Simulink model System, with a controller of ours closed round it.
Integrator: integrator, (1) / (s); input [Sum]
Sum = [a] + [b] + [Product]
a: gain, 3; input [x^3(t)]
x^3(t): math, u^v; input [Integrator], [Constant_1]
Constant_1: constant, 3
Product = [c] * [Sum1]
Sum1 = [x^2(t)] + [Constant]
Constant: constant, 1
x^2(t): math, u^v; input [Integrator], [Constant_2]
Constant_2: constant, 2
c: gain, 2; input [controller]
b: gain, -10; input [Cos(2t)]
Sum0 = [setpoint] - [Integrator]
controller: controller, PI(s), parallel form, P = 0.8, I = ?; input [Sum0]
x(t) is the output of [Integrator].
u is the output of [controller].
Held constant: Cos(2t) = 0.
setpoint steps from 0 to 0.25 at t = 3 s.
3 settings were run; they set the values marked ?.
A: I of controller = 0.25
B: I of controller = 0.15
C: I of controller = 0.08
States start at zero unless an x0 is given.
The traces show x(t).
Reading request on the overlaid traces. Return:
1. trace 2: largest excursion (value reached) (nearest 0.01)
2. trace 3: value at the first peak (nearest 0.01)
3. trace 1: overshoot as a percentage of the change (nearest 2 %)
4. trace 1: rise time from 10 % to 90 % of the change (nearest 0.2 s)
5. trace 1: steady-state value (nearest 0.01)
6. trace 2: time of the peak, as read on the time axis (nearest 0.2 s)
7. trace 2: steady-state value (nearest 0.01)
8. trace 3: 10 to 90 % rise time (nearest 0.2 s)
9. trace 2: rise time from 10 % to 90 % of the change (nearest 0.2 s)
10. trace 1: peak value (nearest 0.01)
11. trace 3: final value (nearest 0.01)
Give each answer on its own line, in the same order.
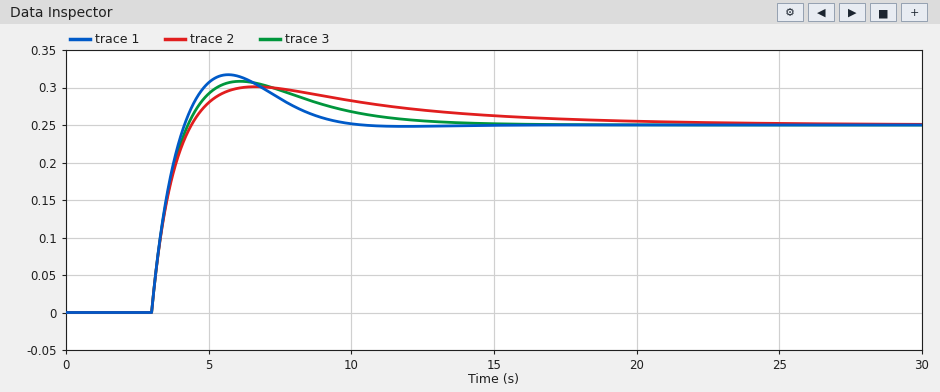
0.30
0.31
26 %
0.8 s
0.25
6.6 s
0.25
1.0 s
1.0 s
0.32
0.25
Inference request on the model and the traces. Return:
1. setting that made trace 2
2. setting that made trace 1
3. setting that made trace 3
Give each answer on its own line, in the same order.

C
A
B
